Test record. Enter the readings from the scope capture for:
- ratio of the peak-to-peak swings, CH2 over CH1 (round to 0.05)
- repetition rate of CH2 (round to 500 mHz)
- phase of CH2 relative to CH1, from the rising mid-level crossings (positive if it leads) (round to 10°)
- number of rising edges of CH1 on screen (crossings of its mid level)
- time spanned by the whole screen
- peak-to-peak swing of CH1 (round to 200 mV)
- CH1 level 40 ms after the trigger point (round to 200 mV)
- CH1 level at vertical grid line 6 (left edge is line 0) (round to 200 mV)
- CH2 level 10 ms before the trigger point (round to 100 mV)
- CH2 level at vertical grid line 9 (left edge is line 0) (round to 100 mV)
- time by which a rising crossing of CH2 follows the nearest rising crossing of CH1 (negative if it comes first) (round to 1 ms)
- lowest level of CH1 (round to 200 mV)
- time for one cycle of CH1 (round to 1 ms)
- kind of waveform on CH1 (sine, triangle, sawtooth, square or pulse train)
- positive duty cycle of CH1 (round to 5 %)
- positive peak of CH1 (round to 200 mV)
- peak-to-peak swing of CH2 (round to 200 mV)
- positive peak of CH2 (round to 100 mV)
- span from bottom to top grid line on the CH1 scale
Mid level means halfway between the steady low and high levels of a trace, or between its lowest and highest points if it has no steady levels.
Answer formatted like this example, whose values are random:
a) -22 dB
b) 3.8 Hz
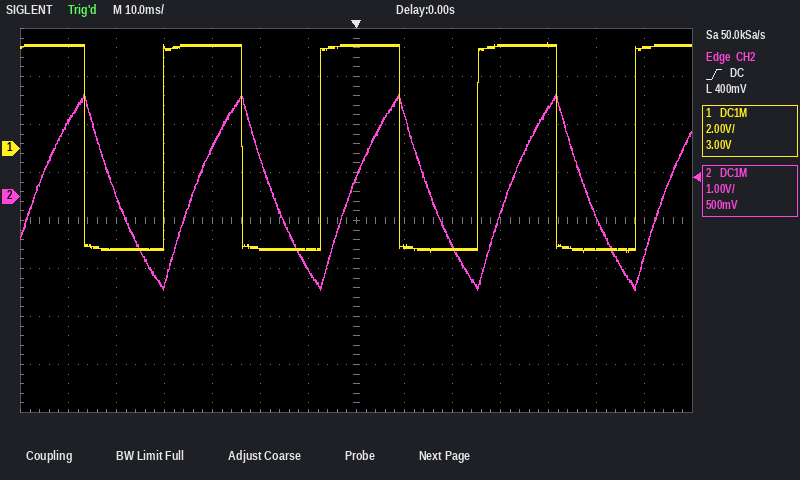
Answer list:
a) 0.45
b) 30.5 Hz
c) -70°
d) 4
e) 140 ms
f) 8.8 V
g) 4.4 V
h) -4.2 V
i) -1.5 V
j) -1.0 V
k) +6 ms
l) -4.4 V
m) 33 ms
n) square
o) 50 %
p) 4.4 V
q) 4.0 V
r) 2.1 V
s) 16 V
